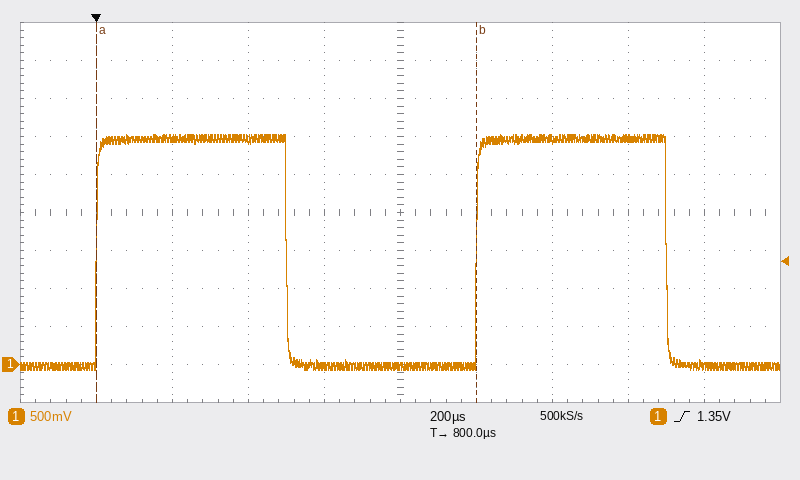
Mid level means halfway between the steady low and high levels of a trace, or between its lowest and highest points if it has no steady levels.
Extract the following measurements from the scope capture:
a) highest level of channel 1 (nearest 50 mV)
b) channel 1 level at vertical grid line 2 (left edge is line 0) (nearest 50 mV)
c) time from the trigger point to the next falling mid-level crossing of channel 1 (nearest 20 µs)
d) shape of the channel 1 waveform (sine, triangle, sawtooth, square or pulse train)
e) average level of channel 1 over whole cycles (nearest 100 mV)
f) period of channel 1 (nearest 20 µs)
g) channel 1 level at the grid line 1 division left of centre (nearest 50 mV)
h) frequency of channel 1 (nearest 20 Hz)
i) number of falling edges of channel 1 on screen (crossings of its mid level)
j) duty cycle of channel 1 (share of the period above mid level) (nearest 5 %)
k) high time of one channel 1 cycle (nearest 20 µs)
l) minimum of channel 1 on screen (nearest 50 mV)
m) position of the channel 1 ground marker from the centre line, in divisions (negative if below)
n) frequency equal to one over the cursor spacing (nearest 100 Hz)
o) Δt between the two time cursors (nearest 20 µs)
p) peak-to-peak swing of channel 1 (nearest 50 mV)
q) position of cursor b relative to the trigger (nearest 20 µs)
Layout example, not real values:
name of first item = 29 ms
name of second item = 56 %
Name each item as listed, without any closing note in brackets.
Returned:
highest level of channel 1 = 3.05 V
channel 1 level at vertical grid line 2 (left edge is line 0) = 3.00 V
time from the trigger point to the next falling mid-level crossing of channel 1 = 500 µs
shape of the channel 1 waveform = square
average level of channel 1 over whole cycles = 1.5 V
period of channel 1 = 1.00 ms
channel 1 level at the grid line 1 division left of centre = 0 mV
frequency of channel 1 = 1.00 kHz
number of falling edges of channel 1 on screen = 2
duty cycle of channel 1 (share of the period above mid level) = 50 %
high time of one channel 1 cycle = 500 µs
minimum of channel 1 on screen = -50 mV
position of the channel 1 ground marker from the centre line, in divisions = -4.0 div
frequency equal to one over the cursor spacing = 1.0 kHz
Δt between the two time cursors = 1.00 ms
peak-to-peak swing of channel 1 = 3.10 V
position of cursor b relative to the trigger = +1.00 ms
